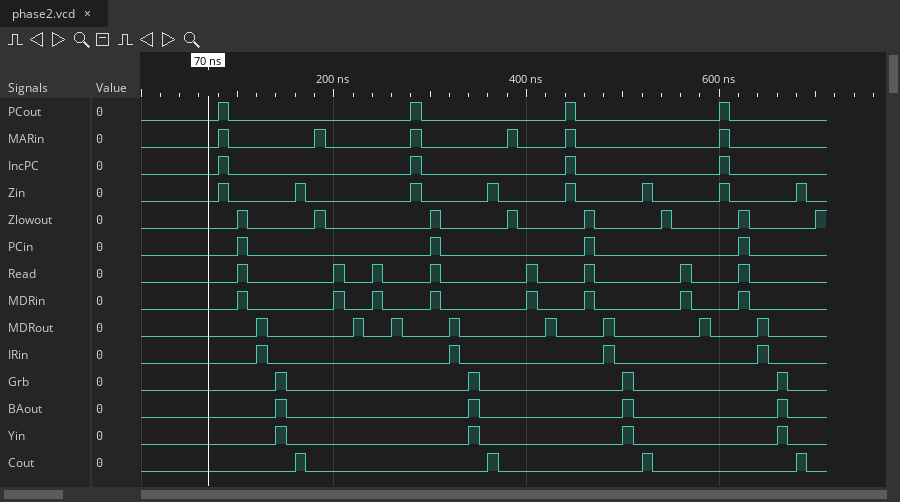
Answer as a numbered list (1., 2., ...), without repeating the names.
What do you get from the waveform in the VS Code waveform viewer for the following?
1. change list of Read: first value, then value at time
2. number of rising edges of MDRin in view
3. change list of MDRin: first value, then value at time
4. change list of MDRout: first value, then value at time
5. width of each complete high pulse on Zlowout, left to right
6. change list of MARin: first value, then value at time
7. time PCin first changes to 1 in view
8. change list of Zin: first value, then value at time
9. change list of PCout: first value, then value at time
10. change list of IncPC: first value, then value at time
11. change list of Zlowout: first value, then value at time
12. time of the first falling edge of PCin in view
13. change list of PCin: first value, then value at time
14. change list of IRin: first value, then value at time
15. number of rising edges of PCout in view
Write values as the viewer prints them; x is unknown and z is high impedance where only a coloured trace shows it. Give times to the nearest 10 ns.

1. 0, 1 at 100 ns, 0 at 110 ns, 1 at 200 ns, 0 at 210 ns, 1 at 240 ns, 0 at 250 ns, 1 at 300 ns, 0 at 310 ns, 1 at 400 ns, 0 at 410 ns, 1 at 460 ns, 0 at 470 ns, 1 at 560 ns, 0 at 570 ns, 1 at 620 ns, 0 at 630 ns
2. 8
3. 0, 1 at 100 ns, 0 at 110 ns, 1 at 200 ns, 0 at 210 ns, 1 at 240 ns, 0 at 250 ns, 1 at 300 ns, 0 at 310 ns, 1 at 400 ns, 0 at 410 ns, 1 at 460 ns, 0 at 470 ns, 1 at 560 ns, 0 at 570 ns, 1 at 620 ns, 0 at 630 ns
4. 0, 1 at 120 ns, 0 at 130 ns, 1 at 220 ns, 0 at 230 ns, 1 at 260 ns, 0 at 270 ns, 1 at 320 ns, 0 at 330 ns, 1 at 420 ns, 0 at 430 ns, 1 at 480 ns, 0 at 490 ns, 1 at 580 ns, 0 at 590 ns, 1 at 640 ns, 0 at 650 ns
5. 10 ns, 10 ns, 10 ns, 10 ns, 10 ns, 10 ns, 10 ns
6. 0, 1 at 80 ns, 0 at 90 ns, 1 at 180 ns, 0 at 190 ns, 1 at 280 ns, 0 at 290 ns, 1 at 380 ns, 0 at 390 ns, 1 at 440 ns, 0 at 450 ns, 1 at 600 ns, 0 at 610 ns
7. 100 ns
8. 0, 1 at 80 ns, 0 at 90 ns, 1 at 160 ns, 0 at 170 ns, 1 at 280 ns, 0 at 290 ns, 1 at 360 ns, 0 at 370 ns, 1 at 440 ns, 0 at 450 ns, 1 at 520 ns, 0 at 530 ns, 1 at 600 ns, 0 at 610 ns, 1 at 680 ns, 0 at 690 ns
9. 0, 1 at 80 ns, 0 at 90 ns, 1 at 280 ns, 0 at 290 ns, 1 at 440 ns, 0 at 450 ns, 1 at 600 ns, 0 at 610 ns
10. 0, 1 at 80 ns, 0 at 90 ns, 1 at 280 ns, 0 at 290 ns, 1 at 440 ns, 0 at 450 ns, 1 at 600 ns, 0 at 610 ns
11. 0, 1 at 100 ns, 0 at 110 ns, 1 at 180 ns, 0 at 190 ns, 1 at 300 ns, 0 at 310 ns, 1 at 380 ns, 0 at 390 ns, 1 at 460 ns, 0 at 470 ns, 1 at 540 ns, 0 at 550 ns, 1 at 620 ns, 0 at 630 ns, 1 at 700 ns
12. 110 ns
13. 0, 1 at 100 ns, 0 at 110 ns, 1 at 300 ns, 0 at 310 ns, 1 at 460 ns, 0 at 470 ns, 1 at 620 ns, 0 at 630 ns
14. 0, 1 at 120 ns, 0 at 130 ns, 1 at 320 ns, 0 at 330 ns, 1 at 480 ns, 0 at 490 ns, 1 at 640 ns, 0 at 650 ns
15. 4
